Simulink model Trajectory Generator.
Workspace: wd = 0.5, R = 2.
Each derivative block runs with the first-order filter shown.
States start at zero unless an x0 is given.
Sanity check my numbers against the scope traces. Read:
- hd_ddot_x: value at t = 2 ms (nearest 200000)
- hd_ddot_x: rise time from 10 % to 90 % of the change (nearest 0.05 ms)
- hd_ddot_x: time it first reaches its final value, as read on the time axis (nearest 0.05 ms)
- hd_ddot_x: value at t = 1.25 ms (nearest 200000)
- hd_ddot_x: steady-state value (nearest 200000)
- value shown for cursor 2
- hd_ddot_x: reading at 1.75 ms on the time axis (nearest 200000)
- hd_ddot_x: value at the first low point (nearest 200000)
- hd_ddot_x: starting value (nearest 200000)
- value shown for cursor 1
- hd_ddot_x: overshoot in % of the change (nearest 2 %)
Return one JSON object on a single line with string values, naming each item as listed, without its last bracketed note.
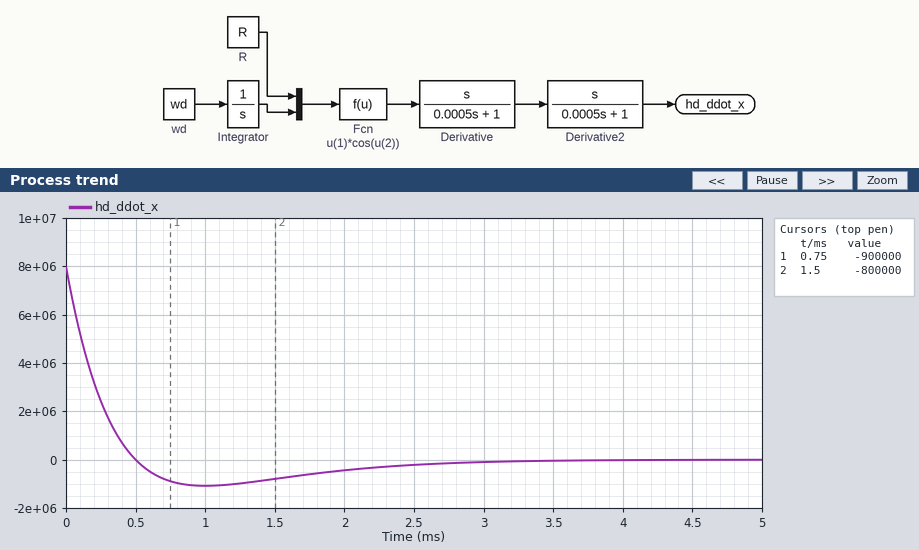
{"hd_ddot_x: value at t = 2 ms": "-400000", "hd_ddot_x: rise time from 10 % to 90 % of the change": "0.35 ms", "hd_ddot_x: time it first reaches its final value, as read on the time axis": "0.50 ms", "hd_ddot_x: value at t = 1.25 ms": "-1000000", "hd_ddot_x: steady-state value": "0", "value shown for cursor 2": "-800000", "hd_ddot_x: reading at 1.75 ms on the time axis": "-600000", "hd_ddot_x: value at the first low point": "-1000000", "hd_ddot_x: starting value": "8000000", "value shown for cursor 1": "-900000", "hd_ddot_x: overshoot in % of the change": "14 %"}
